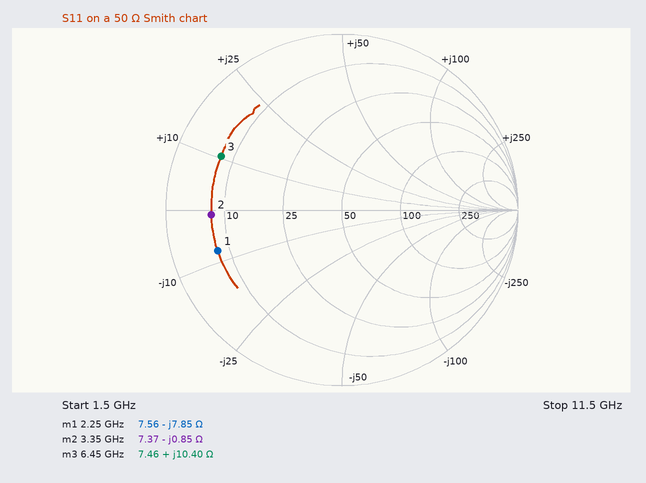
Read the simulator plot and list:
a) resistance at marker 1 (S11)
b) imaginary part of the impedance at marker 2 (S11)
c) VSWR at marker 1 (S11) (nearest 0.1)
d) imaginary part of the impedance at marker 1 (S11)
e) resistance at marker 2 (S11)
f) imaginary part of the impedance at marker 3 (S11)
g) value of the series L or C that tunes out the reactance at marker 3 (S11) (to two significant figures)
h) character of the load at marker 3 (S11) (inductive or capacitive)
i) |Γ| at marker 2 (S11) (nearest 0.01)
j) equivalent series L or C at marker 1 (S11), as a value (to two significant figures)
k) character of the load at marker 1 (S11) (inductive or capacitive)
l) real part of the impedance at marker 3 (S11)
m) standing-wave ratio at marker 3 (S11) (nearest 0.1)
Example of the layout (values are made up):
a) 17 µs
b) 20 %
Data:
a) 7.56 Ω
b) -0.85 Ω
c) 6.8
d) -7.85 Ω
e) 7.37 Ω
f) +10.40 Ω
g) 2.4 pF
h) inductive
i) 0.74
j) 9.0 pF
k) capacitive
l) 7.46 Ω
m) 7.0
